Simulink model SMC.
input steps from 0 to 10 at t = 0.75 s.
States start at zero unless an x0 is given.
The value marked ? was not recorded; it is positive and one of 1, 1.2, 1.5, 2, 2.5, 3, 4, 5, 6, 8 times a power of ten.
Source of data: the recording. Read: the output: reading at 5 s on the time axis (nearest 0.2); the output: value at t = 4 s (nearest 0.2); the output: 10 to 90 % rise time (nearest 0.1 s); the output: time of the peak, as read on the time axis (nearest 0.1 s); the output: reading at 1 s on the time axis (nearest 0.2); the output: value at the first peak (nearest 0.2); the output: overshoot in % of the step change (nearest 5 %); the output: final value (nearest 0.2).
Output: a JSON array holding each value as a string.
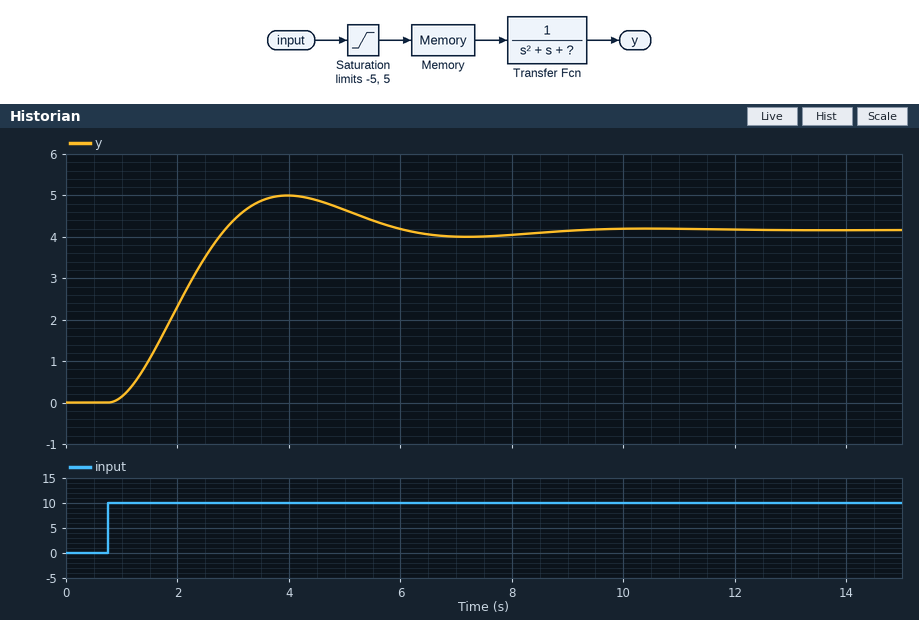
["4.6", "5.0", "1.4 s", "4.0 s", "0.2", "5.0", "20 %", "4.2"]
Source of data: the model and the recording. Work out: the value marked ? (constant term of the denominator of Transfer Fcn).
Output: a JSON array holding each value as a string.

["1.2"]
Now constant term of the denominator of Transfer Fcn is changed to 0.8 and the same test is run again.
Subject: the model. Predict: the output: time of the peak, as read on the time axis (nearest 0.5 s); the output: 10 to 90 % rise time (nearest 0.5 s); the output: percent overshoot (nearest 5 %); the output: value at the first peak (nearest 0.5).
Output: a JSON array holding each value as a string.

["5.0 s", "2.0 s", "10 %", "7.0"]
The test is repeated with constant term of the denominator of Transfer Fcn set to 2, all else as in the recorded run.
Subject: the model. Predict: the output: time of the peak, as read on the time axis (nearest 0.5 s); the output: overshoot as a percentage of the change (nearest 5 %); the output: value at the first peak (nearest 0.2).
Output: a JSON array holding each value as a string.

["3.0 s", "30 %", "3.2"]
